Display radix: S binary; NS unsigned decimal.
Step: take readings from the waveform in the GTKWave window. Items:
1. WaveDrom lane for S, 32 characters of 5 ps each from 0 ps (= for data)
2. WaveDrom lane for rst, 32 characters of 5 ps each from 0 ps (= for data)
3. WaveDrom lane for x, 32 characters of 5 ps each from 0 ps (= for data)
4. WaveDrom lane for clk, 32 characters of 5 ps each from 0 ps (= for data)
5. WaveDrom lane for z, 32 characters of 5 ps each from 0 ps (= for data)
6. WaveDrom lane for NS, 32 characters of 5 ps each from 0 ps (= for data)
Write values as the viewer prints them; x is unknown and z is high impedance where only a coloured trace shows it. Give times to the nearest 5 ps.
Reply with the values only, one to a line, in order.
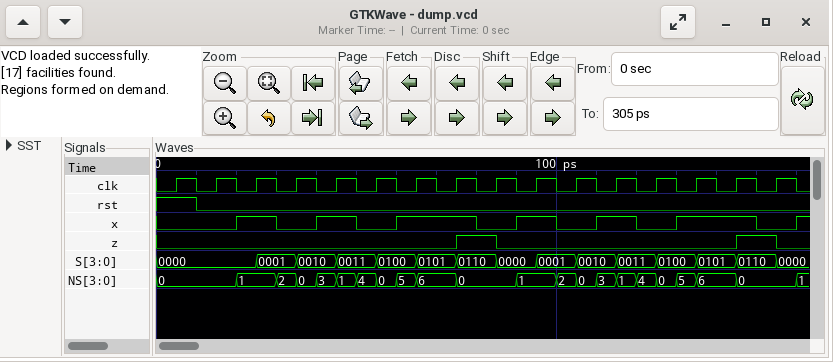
{name: 'S', wave: '=....=.=.=.=.=.=.=.=.=.=.=.=.=.=', data: '0000 0001 0010 0011 0100 0101 0110 0000 0001 0010 0011 0100 0101 0110 0000'}
{name: 'rst', wave: '1.0.............................'}
{name: 'x', wave: '0...1.0.1.0.1...0.1.0.1.0.1...0.'}
{name: 'clk', wave: '01010101010101010101010101010101'}
{name: 'z', wave: '0..............1.0...........1.0'}
{name: 'NS', wave: '=...=.========.=..=.========.=..', data: '0 1 2 0 3 1 4 0 5 6 0 1 2 0 3 1 4 0 5 6 0'}
